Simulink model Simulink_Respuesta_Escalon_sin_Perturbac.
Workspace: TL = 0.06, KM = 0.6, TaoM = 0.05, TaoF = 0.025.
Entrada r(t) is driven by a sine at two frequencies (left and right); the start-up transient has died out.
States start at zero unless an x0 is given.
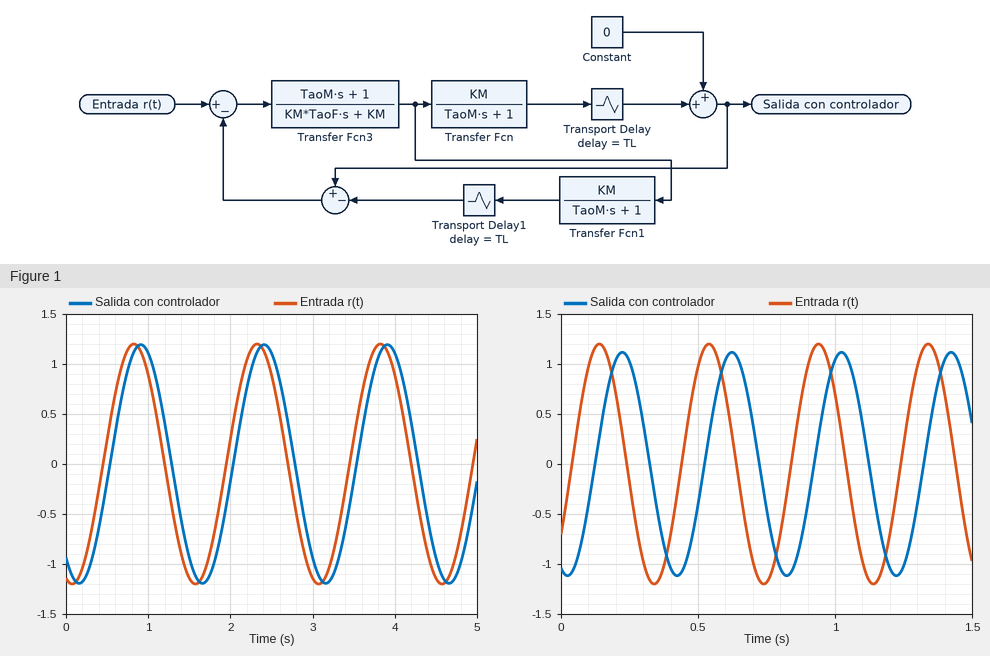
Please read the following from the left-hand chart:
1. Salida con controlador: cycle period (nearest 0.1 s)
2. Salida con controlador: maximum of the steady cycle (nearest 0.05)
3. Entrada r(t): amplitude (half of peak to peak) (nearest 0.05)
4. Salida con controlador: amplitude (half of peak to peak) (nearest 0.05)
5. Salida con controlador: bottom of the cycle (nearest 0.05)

1.5 s
1.20
1.20
1.20
-1.20
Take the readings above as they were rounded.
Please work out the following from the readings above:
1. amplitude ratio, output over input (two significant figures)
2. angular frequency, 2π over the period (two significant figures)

1.0
4.2 rad/s
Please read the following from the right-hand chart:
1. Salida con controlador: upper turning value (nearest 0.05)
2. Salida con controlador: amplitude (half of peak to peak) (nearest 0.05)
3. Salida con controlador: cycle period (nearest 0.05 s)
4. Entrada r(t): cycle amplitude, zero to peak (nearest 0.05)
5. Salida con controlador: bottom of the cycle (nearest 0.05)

1.10
1.10
0.40 s
1.20
-1.10
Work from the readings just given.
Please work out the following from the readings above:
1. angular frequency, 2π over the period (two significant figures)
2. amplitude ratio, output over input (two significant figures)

16 rad/s
0.92
